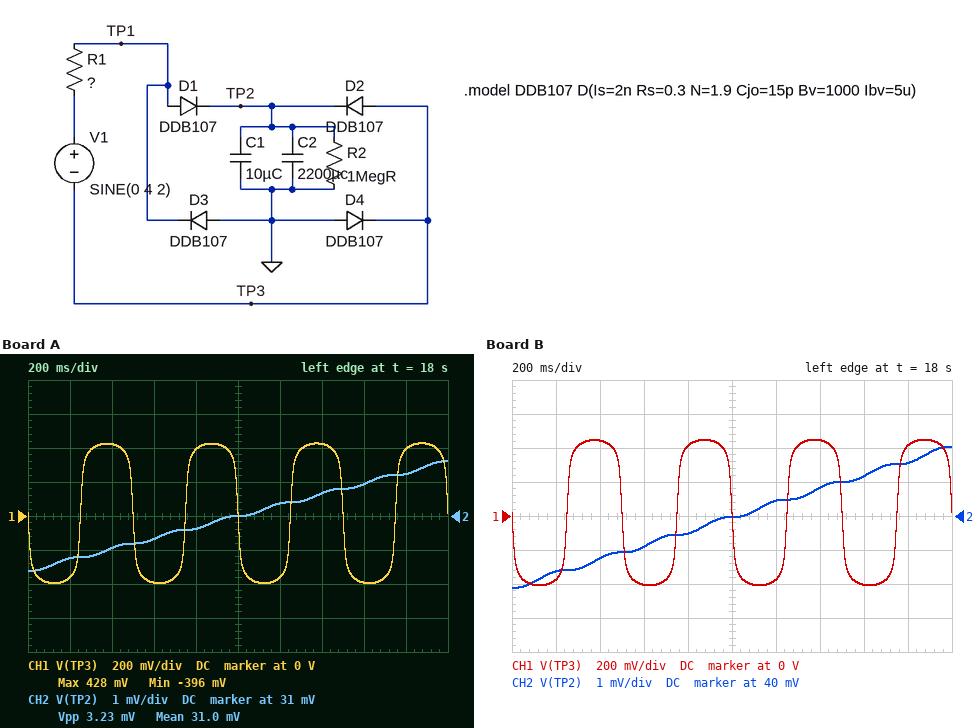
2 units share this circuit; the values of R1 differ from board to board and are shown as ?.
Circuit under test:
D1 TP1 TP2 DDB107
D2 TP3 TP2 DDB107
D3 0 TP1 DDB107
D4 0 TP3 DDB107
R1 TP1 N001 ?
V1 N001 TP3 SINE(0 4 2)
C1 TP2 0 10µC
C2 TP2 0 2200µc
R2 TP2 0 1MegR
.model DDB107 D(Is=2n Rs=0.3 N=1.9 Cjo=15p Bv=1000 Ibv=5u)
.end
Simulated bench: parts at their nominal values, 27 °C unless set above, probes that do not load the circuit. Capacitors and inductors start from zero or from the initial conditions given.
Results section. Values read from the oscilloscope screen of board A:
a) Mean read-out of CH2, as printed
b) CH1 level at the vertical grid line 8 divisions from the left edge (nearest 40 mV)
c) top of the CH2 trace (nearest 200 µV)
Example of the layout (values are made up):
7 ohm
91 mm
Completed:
31.0 mV
-400 mV
32.6 mV
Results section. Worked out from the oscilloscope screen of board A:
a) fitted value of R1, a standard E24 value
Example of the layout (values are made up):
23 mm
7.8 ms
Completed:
510 kΩ
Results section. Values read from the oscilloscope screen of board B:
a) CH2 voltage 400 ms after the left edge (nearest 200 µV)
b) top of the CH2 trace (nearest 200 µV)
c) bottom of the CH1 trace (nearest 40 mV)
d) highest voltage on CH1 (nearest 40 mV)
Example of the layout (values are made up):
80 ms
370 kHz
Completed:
38.8 mV
42.0 mV
-400 mV
440 mV
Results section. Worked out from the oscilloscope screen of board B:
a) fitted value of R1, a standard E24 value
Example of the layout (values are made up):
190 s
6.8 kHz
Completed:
390 kΩ
